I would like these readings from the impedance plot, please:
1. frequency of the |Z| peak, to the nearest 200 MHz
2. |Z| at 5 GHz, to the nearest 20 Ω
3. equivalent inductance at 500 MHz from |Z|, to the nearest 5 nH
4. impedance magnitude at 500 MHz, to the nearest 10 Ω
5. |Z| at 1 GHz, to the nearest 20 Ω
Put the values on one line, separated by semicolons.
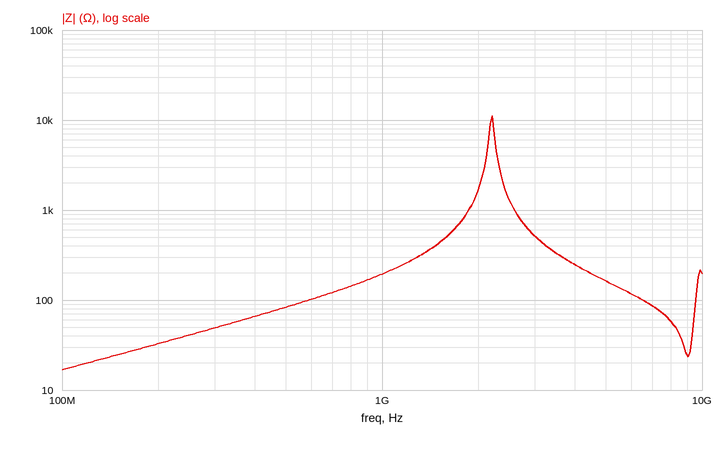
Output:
2.2 GHz; 160 Ω; 25 nH; 80 Ω; 200 Ω
